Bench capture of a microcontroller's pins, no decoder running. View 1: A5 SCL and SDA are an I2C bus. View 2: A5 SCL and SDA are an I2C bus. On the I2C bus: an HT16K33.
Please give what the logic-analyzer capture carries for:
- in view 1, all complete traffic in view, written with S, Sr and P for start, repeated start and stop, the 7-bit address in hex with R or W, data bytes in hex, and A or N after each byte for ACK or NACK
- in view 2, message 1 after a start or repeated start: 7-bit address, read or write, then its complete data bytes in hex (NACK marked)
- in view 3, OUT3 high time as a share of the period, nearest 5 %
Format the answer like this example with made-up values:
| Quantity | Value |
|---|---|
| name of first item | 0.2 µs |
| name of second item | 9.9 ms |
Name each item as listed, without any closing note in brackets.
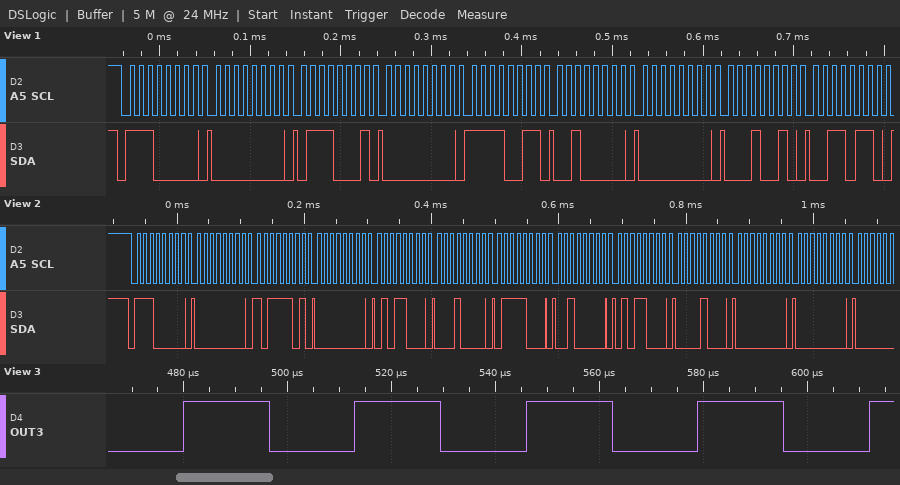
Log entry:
| Quantity | Value |
|---|---|
| in view 1, all complete traffic in view, written with S, Sr and P for start, repeated start and stop, the 7-bit address in hex with R or W, data bytes in hex, and A or N after each byte for ACK or NACK | S 70W A 00 A 71 A 00 A F3 A 20 A 00 A 12 A 36 A |
| in view 2, message 1 after a start or repeated start: 7-bit address, read or write, then its complete data bytes in hex | 0x70 write: 00 BD 00 58 10 78 20 58 08 00 00 |
| in view 3, OUT3 high time as a share of the period, nearest 5 % | 50 % |
